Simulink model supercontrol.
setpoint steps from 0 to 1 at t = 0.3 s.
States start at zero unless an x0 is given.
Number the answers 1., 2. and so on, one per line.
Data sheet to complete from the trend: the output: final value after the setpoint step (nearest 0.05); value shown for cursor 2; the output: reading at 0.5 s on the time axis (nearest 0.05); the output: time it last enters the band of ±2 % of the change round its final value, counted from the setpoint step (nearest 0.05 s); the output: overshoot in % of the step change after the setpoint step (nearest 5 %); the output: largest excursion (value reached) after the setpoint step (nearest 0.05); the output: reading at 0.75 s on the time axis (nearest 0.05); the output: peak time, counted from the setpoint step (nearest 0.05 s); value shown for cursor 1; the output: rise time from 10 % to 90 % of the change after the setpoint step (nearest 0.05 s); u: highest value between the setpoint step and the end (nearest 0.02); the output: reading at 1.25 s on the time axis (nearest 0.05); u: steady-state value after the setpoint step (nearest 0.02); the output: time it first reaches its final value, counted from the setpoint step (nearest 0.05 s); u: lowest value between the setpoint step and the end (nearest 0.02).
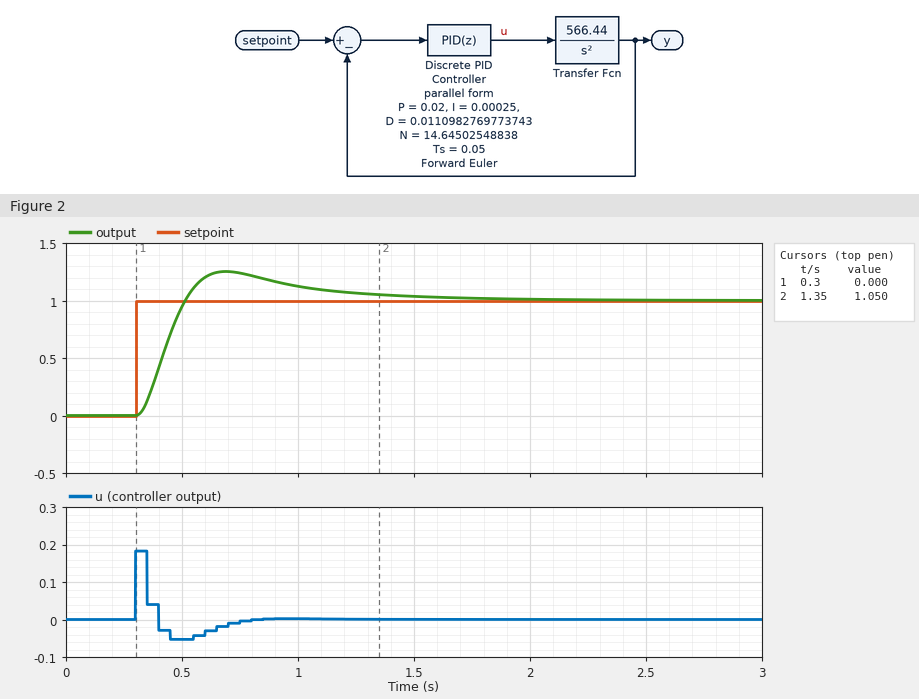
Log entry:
1. 1.00
2. 1.050
3. 0.95
4. 1.45 s
5. 25 %
6. 1.25
7. 1.25
8. 0.40 s
9. 0.000
10. 0.15 s
11. 0.18
12. 1.05
13. 0.00
14. 0.20 s
15. -0.06
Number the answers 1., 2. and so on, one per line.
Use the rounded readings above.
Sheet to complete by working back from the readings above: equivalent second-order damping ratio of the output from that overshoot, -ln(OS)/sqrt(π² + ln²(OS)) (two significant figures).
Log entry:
1. 0.40
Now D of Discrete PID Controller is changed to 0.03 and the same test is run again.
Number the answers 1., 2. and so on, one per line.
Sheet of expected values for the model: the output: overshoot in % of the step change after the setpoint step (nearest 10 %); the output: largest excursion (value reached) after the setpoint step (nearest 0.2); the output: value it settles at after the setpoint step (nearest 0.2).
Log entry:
1. 50 %
2. 1.4
3. 1.0
